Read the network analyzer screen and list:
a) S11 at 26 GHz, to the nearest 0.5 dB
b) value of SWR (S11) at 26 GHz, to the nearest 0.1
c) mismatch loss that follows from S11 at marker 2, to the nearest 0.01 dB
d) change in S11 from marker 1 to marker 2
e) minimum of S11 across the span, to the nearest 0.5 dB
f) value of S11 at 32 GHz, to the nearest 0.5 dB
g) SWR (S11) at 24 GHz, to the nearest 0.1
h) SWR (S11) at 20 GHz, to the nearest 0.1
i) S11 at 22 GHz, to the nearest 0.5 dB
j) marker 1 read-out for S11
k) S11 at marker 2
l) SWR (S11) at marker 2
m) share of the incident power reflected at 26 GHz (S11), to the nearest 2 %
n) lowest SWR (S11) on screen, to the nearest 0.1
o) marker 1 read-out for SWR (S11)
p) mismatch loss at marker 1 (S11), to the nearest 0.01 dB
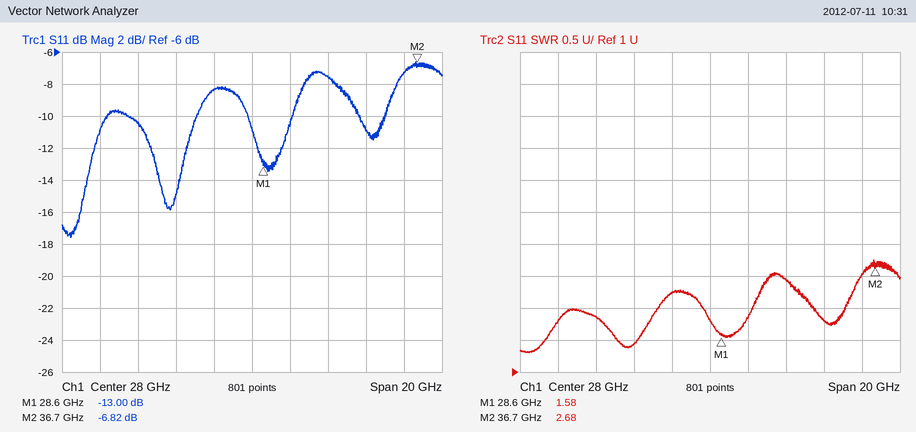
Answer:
-8.5 dB
2.2
1.01 dB
6.18 dB
-17.5 dB
-7.5 dB
1.4
1.8
-10.5 dB
-13.00 dB
-6.82 dB
2.68
14 %
1.3
1.58
0.22 dB
